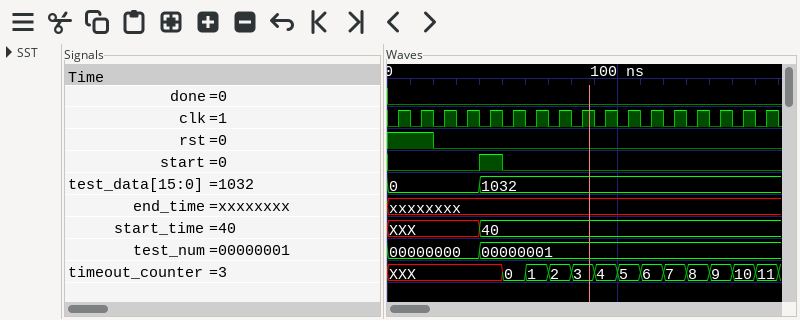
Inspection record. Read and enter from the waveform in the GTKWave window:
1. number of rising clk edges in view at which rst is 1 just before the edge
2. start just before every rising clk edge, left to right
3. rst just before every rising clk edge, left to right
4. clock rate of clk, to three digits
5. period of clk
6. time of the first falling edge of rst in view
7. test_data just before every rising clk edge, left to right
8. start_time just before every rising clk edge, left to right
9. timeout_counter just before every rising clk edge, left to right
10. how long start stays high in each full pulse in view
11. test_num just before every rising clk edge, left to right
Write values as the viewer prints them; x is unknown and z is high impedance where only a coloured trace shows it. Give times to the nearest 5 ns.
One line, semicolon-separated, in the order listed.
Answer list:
2; 0 0 0 0 1 0 0 0 0 0 0 0 0 0 0 0 0; 1 1 0 0 0 0 0 0 0 0 0 0 0 0 0 0 0; 100 MHz; 10 ns; 20 ns; 0, 0, 0, 0, 1032, 1032, 1032, 1032, 1032, 1032, 1032, 1032, 1032, 1032, 1032, 1032, 1032; XXX, XXX, XXX, XXX, 40, 40, 40, 40, 40, 40, 40, 40, 40, 40, 40, 40, 40; XXX, XXX, XXX, XXX, XXX, 0, 1, 2, 3, 4, 5, 6, 7, 8, 9, 10, 11; 10 ns; 00000000, 00000000, 00000000, 00000000, 00000001, 00000001, 00000001, 00000001, 00000001, 00000001, 00000001, 00000001, 00000001, 00000001, 00000001, 00000001, 00000001
